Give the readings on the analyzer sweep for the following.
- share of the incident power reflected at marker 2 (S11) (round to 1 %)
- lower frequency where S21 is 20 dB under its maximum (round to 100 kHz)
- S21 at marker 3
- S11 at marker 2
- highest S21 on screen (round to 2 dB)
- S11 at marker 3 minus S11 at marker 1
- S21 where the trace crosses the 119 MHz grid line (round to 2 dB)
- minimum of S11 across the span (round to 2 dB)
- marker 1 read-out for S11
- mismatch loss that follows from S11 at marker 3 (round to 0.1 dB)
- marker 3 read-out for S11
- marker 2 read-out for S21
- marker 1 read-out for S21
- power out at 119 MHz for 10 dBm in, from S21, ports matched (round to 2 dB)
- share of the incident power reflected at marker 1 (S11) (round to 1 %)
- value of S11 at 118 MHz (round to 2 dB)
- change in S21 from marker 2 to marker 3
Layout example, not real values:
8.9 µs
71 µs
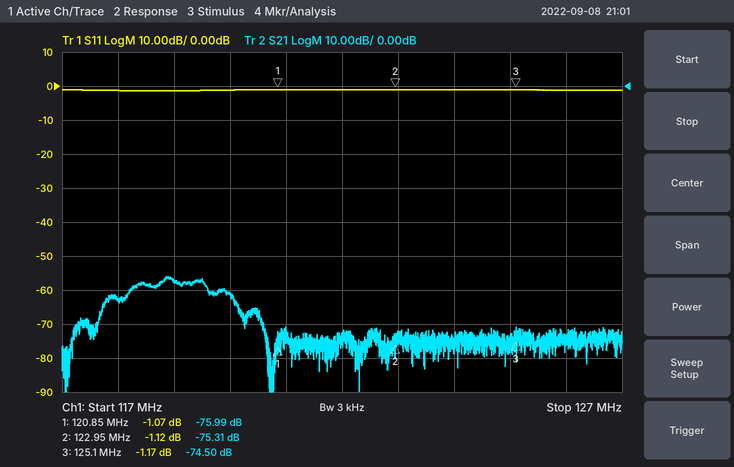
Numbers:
77 %
117.2 MHz
-74.50 dB
-1.12 dB
-56 dB
-0.10 dB
-58 dB
-2 dB
-1.07 dB
6.3 dB
-1.17 dB
-75.31 dB
-75.99 dB
-48 dBm
78 %
-2 dB
0.81 dB
